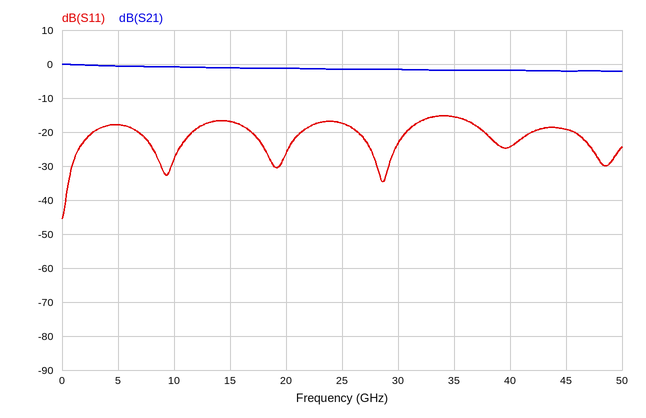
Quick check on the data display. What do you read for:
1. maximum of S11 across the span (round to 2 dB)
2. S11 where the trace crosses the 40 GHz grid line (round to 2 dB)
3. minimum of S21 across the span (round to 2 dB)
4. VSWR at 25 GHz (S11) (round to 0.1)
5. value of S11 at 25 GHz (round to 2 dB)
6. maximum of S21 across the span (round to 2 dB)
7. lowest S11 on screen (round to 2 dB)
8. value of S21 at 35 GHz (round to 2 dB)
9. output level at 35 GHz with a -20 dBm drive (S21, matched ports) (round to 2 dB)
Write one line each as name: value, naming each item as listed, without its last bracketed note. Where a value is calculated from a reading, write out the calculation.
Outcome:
maximum of S11 across the span: -16 dB
S11 where the trace crosses the 40 GHz grid line: -24 dB
minimum of S21 across the span: -2 dB
VSWR at 25 GHz (S11): |Γ| = 10^(-18/20) = 0.1259; VSWR = (1 + 0.1259)/(1 − 0.1259) ≈ 1.3
value of S11 at 25 GHz: -18 dB
maximum of S21 across the span: 0 dB
lowest S11 on screen: -46 dB
value of S21 at 35 GHz: -2 dB
output level at 35 GHz with a -20 dBm drive (S21, matched ports): -20 dBm + (-2 dB) = -22 dBm
